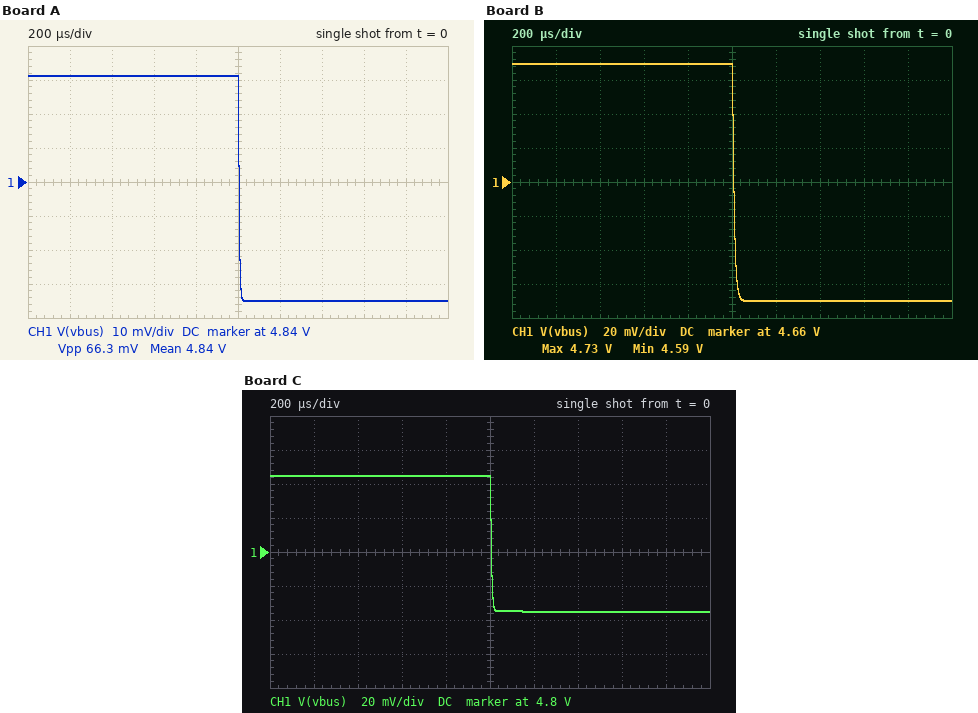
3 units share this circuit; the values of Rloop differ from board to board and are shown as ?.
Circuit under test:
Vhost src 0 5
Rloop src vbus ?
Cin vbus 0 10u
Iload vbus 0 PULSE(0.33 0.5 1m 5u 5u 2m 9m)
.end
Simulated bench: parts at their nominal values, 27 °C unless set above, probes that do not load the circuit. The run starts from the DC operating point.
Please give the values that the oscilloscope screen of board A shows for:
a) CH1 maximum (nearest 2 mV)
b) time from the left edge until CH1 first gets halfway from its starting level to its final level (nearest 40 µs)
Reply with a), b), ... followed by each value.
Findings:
a) 4.872 V
b) 1.00 ms
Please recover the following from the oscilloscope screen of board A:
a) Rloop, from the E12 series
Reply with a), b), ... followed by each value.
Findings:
a) 0.39 Ω
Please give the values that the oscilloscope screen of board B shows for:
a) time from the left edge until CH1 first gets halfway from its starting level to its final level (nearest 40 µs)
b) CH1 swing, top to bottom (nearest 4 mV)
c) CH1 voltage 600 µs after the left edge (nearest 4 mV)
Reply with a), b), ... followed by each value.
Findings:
a) 1.00 ms
b) 140 mV
c) 4.728 V
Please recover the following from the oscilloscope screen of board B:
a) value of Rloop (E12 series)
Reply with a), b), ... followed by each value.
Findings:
a) 0.82 Ω
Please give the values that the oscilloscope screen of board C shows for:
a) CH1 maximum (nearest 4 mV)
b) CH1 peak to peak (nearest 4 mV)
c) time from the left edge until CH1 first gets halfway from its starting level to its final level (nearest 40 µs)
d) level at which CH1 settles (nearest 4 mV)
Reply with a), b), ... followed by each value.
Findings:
a) 4.844 V
b) 80 mV
c) 1.00 ms
d) 4.764 V
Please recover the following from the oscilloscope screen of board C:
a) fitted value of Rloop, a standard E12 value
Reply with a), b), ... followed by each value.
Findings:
a) 0.47 Ω
